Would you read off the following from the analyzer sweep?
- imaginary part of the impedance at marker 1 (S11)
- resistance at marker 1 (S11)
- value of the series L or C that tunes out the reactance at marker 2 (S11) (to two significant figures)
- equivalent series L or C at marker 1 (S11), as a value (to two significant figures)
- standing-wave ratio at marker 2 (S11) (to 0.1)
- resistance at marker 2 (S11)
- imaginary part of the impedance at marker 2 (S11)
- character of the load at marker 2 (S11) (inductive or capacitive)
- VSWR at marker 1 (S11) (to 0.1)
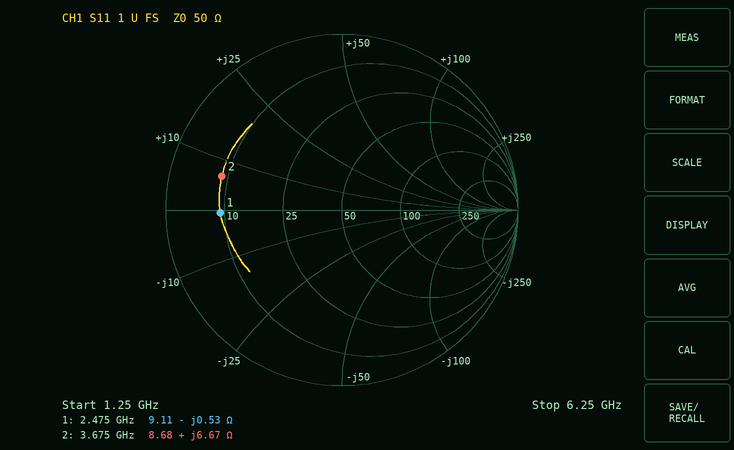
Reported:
-0.53 Ω
9.11 Ω
6.5 pF
120 pF
5.9
8.68 Ω
+6.67 Ω
inductive
5.5
